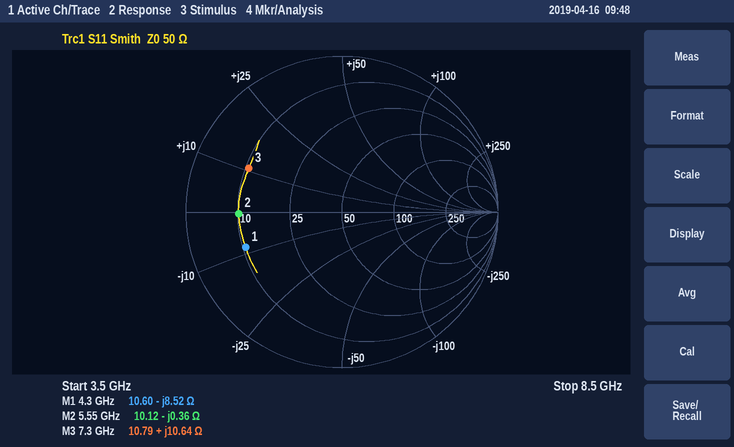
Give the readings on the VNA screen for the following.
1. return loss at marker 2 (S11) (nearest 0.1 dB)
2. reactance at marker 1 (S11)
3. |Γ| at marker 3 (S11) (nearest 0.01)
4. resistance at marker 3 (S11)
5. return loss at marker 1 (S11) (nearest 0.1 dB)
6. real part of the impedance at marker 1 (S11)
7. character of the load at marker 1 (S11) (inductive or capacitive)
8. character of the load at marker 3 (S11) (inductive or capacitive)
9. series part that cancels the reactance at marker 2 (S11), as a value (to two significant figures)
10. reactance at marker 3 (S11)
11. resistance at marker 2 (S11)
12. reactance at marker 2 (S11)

3.6 dB
-8.52 Ω
0.66
10.79 Ω
3.6 dB
10.60 Ω
capacitive
inductive
10 pH
+10.64 Ω
10.12 Ω
-0.36 Ω
